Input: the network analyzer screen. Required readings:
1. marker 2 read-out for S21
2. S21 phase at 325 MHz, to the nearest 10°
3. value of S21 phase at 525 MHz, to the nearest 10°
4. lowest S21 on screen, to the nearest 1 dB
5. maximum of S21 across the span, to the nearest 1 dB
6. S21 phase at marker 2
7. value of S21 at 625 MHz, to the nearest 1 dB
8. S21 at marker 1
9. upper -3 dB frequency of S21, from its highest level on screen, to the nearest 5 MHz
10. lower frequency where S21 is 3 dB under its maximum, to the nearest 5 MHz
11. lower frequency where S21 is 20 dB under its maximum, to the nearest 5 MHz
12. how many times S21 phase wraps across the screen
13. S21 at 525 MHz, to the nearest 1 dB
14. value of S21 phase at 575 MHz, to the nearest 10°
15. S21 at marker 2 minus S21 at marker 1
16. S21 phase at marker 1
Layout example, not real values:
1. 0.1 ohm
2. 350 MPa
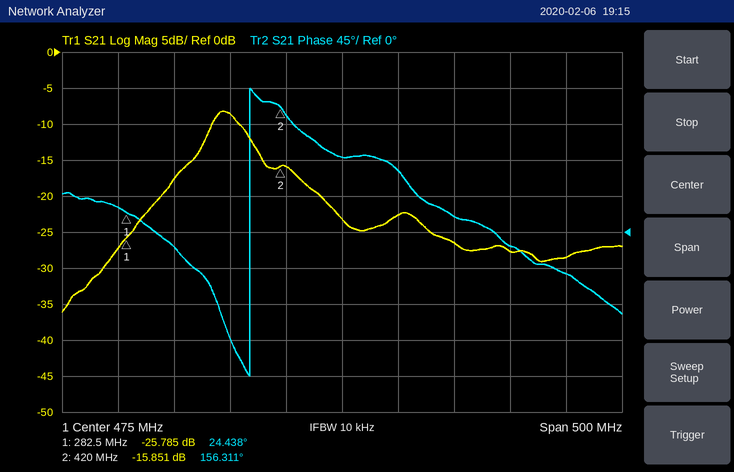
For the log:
1. -15.851 dB
2. -20°
3. 80°
4. -36 dB
5. -8 dB
6. 156.311°
7. -28 dB
8. -25.785 dB
9. 390 MHz
10. 355 MHz
11. 270 MHz
12. 1
13. -23 dB
14. 20°
15. 9.934 dB
16. 24.438°
